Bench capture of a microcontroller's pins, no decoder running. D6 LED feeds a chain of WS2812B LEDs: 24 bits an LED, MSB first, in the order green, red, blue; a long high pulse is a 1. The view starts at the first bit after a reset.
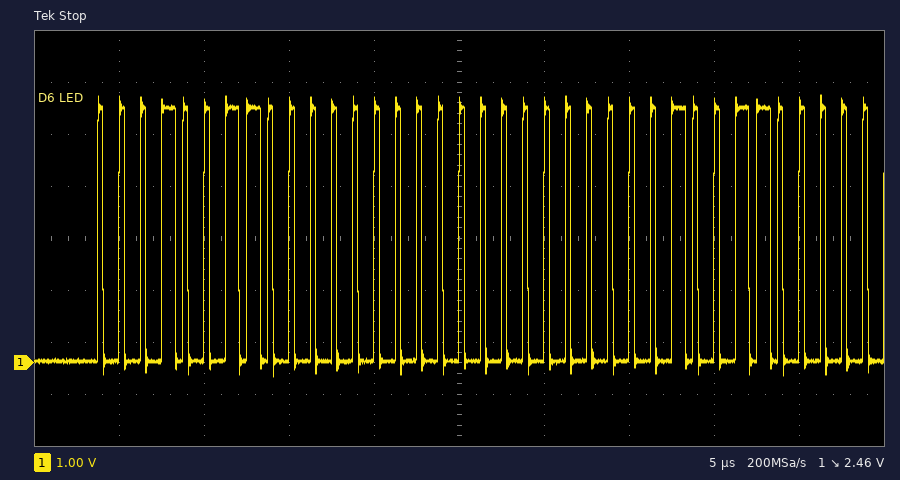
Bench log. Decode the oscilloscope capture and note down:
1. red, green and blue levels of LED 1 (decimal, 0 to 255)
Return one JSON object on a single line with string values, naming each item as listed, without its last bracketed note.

{"red, green and blue levels of LED 1": "0, 19, 0"}
